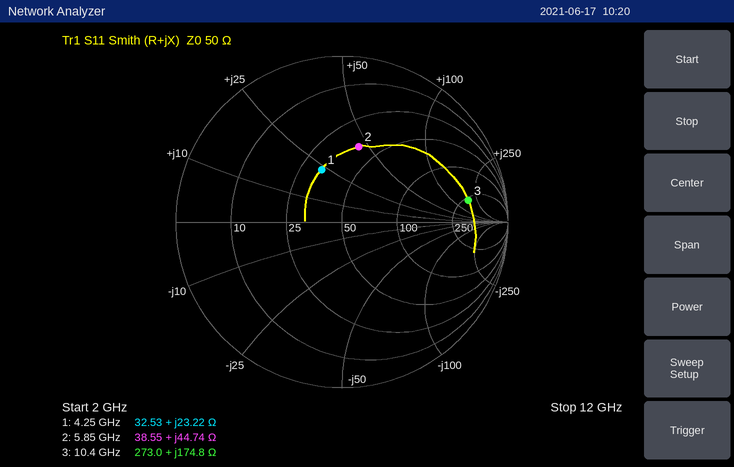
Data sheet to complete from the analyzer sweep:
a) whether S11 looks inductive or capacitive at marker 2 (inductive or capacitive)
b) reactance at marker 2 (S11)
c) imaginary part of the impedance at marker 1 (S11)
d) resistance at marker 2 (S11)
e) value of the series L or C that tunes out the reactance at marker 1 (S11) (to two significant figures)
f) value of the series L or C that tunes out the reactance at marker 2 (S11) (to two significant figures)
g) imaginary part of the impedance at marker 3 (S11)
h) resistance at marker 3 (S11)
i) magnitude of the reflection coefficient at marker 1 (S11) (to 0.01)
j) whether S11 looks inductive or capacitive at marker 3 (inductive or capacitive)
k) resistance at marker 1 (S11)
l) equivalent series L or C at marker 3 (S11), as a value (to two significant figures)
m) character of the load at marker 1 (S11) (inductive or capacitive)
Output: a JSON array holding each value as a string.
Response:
["inductive", "+44.74 Ω", "+23.22 Ω", "38.55 Ω", "1.6 pF", "610 fF", "+174.8 Ω", "273.0 Ω", "0.34", "inductive", "32.53 Ω", "2.7 nH", "inductive"]
